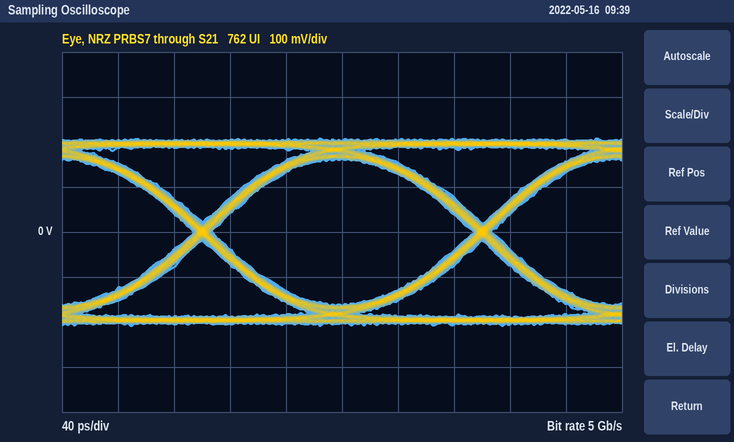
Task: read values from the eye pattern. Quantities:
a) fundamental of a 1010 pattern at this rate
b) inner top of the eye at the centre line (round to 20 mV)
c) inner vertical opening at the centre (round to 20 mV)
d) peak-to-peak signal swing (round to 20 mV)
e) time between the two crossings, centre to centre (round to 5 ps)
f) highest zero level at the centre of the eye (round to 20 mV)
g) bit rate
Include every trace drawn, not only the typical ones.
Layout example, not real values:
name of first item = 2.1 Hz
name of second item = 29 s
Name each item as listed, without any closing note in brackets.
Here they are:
fundamental of a 1010 pattern at this rate = 2.5 GHz
inner top of the eye at the centre line = 160 mV
inner vertical opening at the centre = 320 mV
peak-to-peak signal swing = 420 mV
time between the two crossings, centre to centre = 200 ps
highest zero level at the centre of the eye = -160 mV
bit rate = 5 Gb/s
